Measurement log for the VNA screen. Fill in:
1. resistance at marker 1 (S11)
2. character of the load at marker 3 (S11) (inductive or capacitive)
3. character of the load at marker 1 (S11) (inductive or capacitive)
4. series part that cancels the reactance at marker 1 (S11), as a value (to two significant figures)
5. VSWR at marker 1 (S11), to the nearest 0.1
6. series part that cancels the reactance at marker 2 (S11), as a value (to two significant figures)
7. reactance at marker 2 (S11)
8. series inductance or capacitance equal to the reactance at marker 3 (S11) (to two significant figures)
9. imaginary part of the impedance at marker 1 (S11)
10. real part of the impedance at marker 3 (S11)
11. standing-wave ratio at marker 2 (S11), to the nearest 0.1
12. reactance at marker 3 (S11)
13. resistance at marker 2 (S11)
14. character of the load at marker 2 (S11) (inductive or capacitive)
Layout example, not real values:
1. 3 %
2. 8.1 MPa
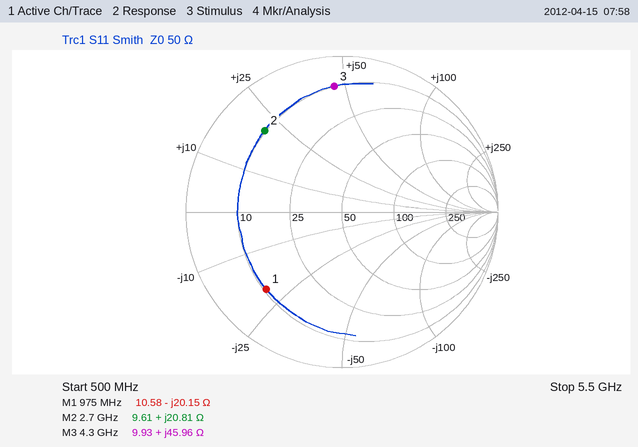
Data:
1. 10.58 Ω
2. inductive
3. capacitive
4. 3.3 nH
5. 5.5
6. 2.8 pF
7. +20.81 Ω
8. 1.7 nH
9. -20.15 Ω
10. 9.93 Ω
11. 6.1
12. +45.96 Ω
13. 9.61 Ω
14. inductive
